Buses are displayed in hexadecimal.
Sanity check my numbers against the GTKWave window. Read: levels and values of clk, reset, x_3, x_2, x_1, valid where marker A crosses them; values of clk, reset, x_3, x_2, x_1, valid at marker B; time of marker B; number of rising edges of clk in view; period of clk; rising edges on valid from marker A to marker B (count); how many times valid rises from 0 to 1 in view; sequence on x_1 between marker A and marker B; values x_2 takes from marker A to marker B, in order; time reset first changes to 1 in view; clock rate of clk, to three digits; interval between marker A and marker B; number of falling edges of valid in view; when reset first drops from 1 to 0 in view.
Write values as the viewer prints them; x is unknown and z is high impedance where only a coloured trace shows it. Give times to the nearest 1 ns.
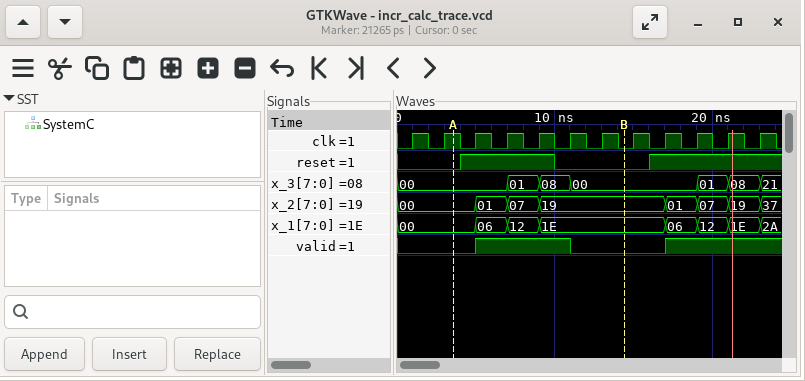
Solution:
clk=1, reset=0, x_3=00, x_2=00, x_1=00, valid=0
clk=0, reset=0, x_3=00, x_2=19, x_1=1E, valid=0
14 ns
12
2 ns
1
2
00, 06, 12, 1E
00, 01, 07, 19
4 ns
500 MHz
11 ns
1
10 ns
